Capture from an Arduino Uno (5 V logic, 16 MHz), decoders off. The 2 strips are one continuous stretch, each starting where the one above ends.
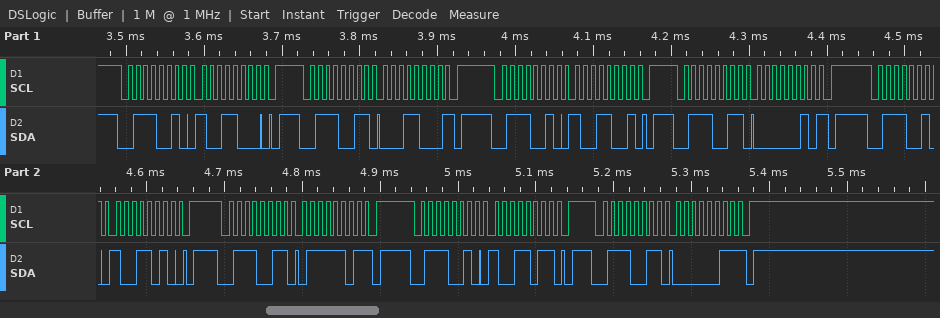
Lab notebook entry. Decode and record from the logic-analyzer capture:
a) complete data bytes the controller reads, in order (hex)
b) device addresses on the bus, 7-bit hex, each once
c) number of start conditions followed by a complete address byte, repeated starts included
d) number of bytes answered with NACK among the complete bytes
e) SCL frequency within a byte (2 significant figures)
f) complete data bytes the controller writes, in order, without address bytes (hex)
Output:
18 02 7D 03
0x39
8
4
100 kHz
98 99 9A 9B
